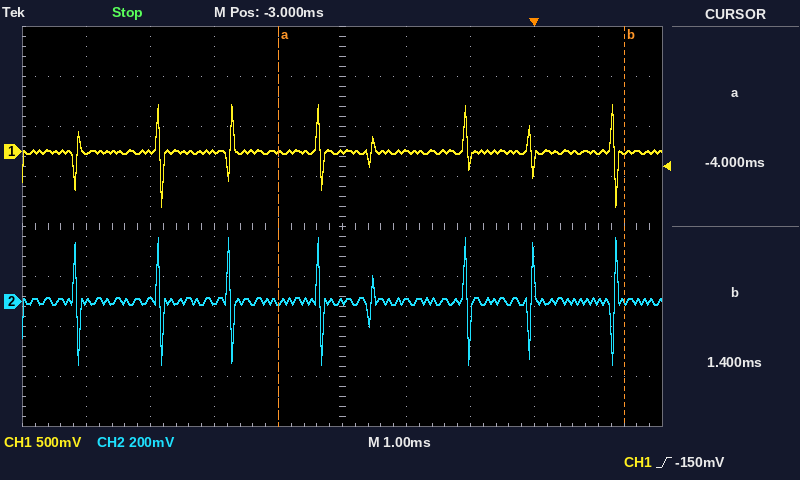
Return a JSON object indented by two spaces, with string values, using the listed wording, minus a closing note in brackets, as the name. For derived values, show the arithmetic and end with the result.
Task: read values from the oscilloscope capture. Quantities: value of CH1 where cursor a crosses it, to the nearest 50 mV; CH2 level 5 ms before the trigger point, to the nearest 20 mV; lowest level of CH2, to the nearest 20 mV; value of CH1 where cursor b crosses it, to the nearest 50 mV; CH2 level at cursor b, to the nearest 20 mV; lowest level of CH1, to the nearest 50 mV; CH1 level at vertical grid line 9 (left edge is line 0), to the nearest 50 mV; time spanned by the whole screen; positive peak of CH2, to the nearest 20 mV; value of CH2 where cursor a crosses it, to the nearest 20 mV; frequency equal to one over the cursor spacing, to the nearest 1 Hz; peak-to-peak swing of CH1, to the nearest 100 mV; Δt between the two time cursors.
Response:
{
  "value of CH1 where cursor a crosses it, to the nearest 50 mV": "0 mV",
  "CH2 level 5 ms before the trigger point, to the nearest 20 mV": "0 mV",
  "lowest level of CH2, to the nearest 20 mV": "-260 mV",
  "value of CH1 where cursor b crosses it, to the nearest 50 mV": "0 mV",
  "CH2 level at cursor b, to the nearest 20 mV": "0 mV",
  "lowest level of CH1, to the nearest 50 mV": "-550 mV",
  "CH1 level at vertical grid line 9 (left edge is line 0), to the nearest 50 mV": "0 mV",
  "time spanned by the whole screen": "10 ms",
  "positive peak of CH2, to the nearest 20 mV": "260 mV",
  "value of CH2 where cursor a crosses it, to the nearest 20 mV": "0 mV",
  "frequency equal to one over the cursor spacing, to the nearest 1 Hz": "1 / 5.4 ms ≈ 185 Hz",
  "peak-to-peak swing of CH1, to the nearest 100 mV": "1.00 V",
  "Δt between the two time cursors": "1.4 ms − (-4 ms) = 5.4 ms"
}
